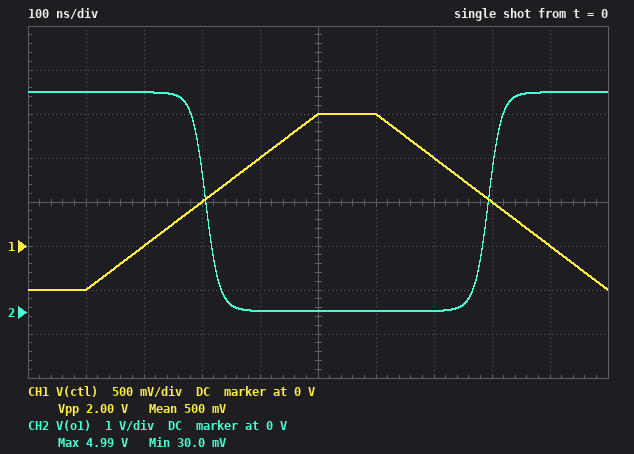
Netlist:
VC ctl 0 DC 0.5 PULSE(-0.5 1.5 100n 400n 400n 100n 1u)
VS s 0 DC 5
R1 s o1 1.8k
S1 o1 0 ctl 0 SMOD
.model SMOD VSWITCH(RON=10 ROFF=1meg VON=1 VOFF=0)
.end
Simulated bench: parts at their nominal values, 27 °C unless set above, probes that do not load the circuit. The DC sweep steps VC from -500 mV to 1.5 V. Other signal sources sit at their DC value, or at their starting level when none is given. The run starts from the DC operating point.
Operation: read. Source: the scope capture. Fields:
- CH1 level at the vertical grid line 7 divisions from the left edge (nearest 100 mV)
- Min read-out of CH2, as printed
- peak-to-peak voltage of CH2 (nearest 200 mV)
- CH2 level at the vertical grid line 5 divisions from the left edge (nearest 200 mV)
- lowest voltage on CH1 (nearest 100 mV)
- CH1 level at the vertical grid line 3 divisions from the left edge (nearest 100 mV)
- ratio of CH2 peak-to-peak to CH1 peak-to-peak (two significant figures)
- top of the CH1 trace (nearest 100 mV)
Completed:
1.0 V
30.0 mV
5.0 V
0 V
-500 mV
500 mV
2.5
1.5 V
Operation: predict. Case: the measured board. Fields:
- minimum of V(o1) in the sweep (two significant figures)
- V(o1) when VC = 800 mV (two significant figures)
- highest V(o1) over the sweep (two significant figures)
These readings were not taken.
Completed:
28 mV
90 mV
5.0 V
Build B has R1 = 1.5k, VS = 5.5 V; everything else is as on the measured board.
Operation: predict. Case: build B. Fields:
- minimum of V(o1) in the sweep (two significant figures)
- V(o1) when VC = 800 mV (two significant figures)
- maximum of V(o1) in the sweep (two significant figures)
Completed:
36 mV
120 mV
5.5 V
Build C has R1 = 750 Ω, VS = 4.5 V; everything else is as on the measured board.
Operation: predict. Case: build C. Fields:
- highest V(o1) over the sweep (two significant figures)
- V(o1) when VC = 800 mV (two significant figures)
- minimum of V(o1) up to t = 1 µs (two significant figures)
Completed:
4.5 V
190 mV
59 mV
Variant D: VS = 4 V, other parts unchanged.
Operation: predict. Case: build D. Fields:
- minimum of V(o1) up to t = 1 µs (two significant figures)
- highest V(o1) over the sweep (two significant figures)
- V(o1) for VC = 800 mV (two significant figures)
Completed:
22 mV
4.0 V
72 mV
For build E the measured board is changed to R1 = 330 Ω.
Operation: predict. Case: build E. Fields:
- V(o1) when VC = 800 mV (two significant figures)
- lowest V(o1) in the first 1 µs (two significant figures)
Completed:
460 mV
150 mV
